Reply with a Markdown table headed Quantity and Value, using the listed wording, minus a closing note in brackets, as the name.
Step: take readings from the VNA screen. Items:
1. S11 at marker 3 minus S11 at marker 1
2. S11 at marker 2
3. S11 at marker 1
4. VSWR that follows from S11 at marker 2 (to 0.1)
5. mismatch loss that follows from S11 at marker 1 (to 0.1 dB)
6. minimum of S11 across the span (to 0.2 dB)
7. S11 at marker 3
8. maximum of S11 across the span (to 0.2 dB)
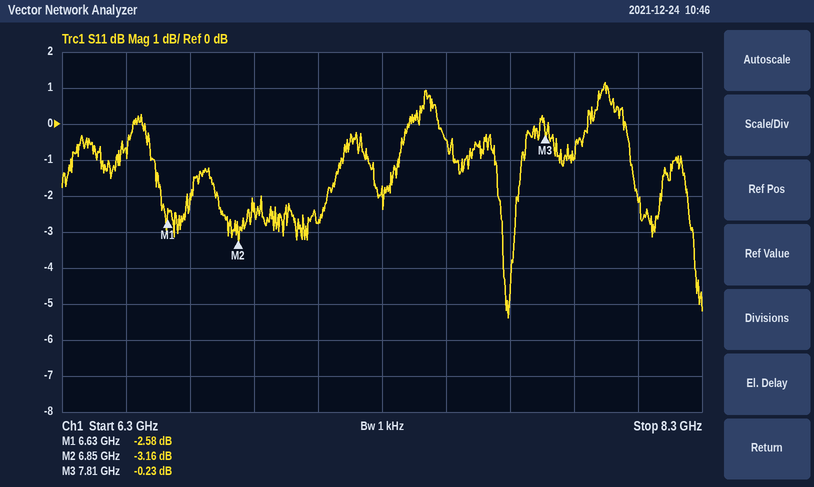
| Quantity | Value |
|---|---|
| S11 at marker 3 minus S11 at marker 1 | 2.35 dB |
| S11 at marker 2 | -3.16 dB |
| S11 at marker 1 | -2.58 dB |
| VSWR that follows from S11 at marker 2 | 5.6 |
| mismatch loss that follows from S11 at marker 1 | 3.5 dB |
| minimum of S11 across the span | -5.4 dB |
| S11 at marker 3 | -0.23 dB |
| maximum of S11 across the span | 1.2 dB |
